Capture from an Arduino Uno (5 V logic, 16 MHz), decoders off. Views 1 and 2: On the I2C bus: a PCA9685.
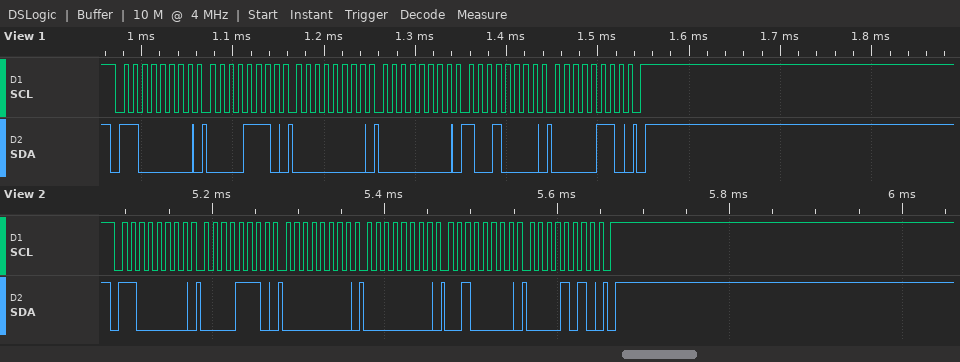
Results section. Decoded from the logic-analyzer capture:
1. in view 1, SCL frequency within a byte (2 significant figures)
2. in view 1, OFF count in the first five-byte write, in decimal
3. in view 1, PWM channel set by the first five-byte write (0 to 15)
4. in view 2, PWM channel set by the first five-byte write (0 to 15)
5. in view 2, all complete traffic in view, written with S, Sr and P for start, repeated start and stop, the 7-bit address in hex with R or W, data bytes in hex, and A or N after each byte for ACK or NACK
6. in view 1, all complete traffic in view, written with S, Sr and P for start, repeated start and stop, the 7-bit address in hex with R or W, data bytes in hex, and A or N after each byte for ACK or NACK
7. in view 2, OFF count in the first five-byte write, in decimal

100 kHz
1680
2
2
S 60W A 0E A 00 A 00 A 20 A 0A A P
S 60W A 0E A 00 A 00 A 90 A 06 A P
2592
